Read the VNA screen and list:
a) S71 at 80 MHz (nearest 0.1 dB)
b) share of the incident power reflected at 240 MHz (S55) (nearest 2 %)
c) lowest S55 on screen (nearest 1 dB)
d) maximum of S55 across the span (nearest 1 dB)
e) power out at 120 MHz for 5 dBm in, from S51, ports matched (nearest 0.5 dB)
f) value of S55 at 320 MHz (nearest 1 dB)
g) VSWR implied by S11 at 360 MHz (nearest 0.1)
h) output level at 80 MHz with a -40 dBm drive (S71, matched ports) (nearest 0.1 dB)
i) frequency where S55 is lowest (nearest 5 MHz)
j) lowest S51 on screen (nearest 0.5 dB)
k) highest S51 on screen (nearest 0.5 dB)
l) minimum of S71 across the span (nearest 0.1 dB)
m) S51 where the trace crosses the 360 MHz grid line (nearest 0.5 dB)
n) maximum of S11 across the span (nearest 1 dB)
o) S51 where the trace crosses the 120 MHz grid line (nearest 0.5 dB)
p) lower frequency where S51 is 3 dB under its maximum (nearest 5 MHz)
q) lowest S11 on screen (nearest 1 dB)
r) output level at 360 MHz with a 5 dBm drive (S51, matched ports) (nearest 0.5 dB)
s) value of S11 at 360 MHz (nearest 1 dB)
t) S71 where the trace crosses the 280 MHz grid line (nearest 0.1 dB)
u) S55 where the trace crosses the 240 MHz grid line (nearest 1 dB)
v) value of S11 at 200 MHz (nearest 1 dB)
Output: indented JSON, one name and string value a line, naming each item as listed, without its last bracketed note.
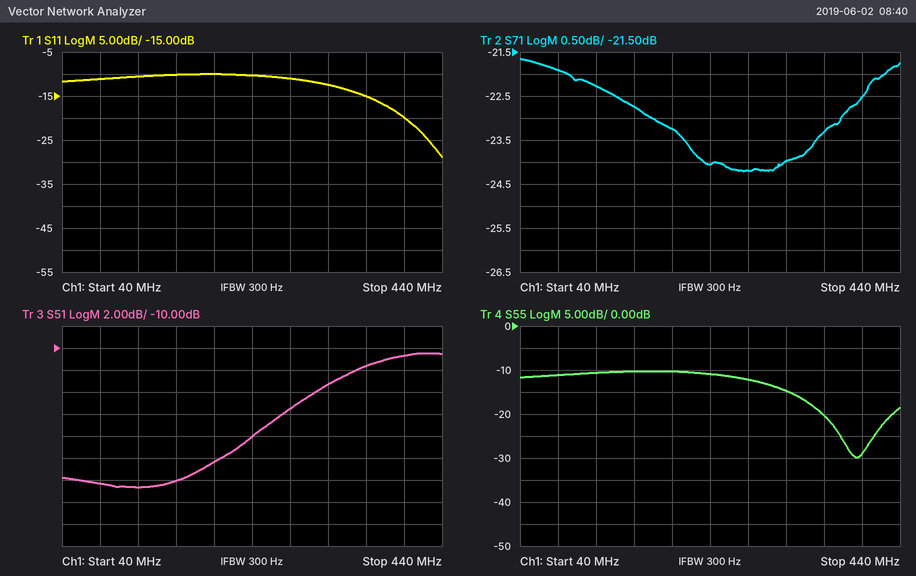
{
  "S71 at 80 MHz": "-21.9 dB",
  "share of the incident power reflected at 240 MHz (S55)": "8 %",
  "lowest S55 on screen": "-30 dB",
  "maximum of S55 across the span": "-10 dB",
  "power out at 120 MHz for 5 dBm in, from S51, ports matched": "-17.5 dBm",
  "value of S55 at 320 MHz": "-15 dB",
  "VSWR implied by S11 at 360 MHz": "1.4",
  "output level at 80 MHz with a -40 dBm drive (S71, matched ports)": "-61.9 dBm",
  "frequency where S55 is lowest": "395 MHz",
  "lowest S51 on screen": "-22.5 dB",
  "highest S51 on screen": "-10.5 dB",
  "minimum of S71 across the span": "-24.2 dB",
  "S51 where the trace crosses the 360 MHz grid line": "-11.5 dB",
  "maximum of S11 across the span": "-10 dB",
  "S51 where the trace crosses the 120 MHz grid line": "-22.5 dB",
  "lower frequency where S51 is 3 dB under its maximum": "315 MHz",
  "lowest S11 on screen": "-29 dB",
  "output level at 360 MHz with a 5 dBm drive (S51, matched ports)": "-6.5 dBm",
  "value of S11 at 360 MHz": "-15 dB",
  "S71 where the trace crosses the 280 MHz grid line": "-24.2 dB",
  "S55 where the trace crosses the 240 MHz grid line": "-11 dB",
  "value of S11 at 200 MHz": "-10 dB"
}
